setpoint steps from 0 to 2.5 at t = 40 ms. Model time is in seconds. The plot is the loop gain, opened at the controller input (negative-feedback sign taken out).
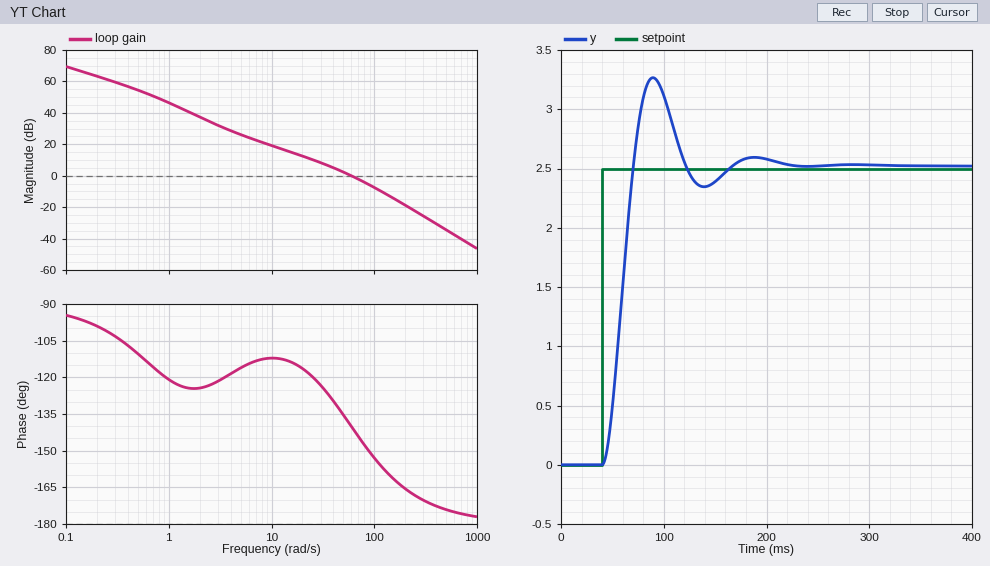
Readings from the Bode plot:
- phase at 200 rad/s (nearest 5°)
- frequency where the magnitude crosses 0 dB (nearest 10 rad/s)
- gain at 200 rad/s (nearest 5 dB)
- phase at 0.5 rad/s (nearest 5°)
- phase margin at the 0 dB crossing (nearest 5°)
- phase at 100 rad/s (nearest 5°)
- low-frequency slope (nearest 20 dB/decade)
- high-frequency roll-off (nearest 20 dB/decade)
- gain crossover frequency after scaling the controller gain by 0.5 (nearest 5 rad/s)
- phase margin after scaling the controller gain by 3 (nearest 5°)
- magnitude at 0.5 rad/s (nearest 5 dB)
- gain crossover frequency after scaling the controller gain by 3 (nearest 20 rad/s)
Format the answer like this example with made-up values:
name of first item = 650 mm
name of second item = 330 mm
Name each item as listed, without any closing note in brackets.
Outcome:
phase at 200 rad/s = -165°
frequency where the magnitude crosses 0 dB = 60 rad/s
gain at 200 rad/s = -20 dB
phase at 0.5 rad/s = -110°
phase margin at the 0 dB crossing = 40°
phase at 100 rad/s = -155°
low-frequency slope = -20 dB/decade
high-frequency roll-off = -40 dB/decade
gain crossover frequency after scaling the controller gain by 0.5 = 35 rad/s
phase margin after scaling the controller gain by 3 = 25°
magnitude at 0.5 rad/s = 55 dB
gain crossover frequency after scaling the controller gain by 3 = 120 rad/s
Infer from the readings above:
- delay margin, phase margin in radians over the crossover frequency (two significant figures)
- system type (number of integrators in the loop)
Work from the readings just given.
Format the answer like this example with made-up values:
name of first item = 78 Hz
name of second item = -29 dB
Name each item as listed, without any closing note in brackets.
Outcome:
delay margin, phase margin in radians over the crossover frequency = 0.012 s
system type = 1
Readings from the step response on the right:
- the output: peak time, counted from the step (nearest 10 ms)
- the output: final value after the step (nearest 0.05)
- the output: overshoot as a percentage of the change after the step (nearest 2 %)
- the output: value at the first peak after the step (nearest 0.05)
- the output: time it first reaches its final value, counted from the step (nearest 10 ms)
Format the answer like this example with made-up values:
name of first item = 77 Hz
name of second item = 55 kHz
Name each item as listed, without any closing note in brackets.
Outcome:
the output: peak time, counted from the step = 50 ms
the output: final value after the step = 2.50
the output: overshoot as a percentage of the change after the step = 30 %
the output: value at the first peak after the step = 3.25
the output: time it first reaches its final value, counted from the step = 30 ms
